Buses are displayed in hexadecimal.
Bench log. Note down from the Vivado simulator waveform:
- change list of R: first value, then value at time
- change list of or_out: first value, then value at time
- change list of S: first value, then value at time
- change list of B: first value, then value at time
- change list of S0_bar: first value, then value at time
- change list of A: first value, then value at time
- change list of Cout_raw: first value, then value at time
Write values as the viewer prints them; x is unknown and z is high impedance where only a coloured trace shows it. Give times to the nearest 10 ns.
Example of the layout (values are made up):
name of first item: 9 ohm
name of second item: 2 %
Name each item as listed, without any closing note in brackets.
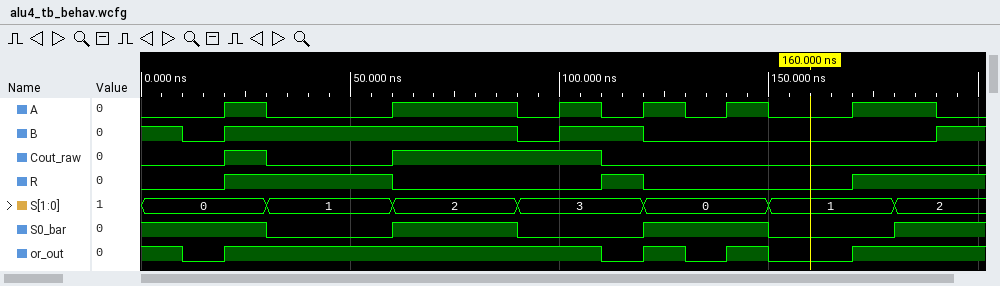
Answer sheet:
change list of R: first value, then value at time: 0, 1 at 20 ns, 0 at 60 ns, 1 at 110 ns, 0 at 120 ns, 1 at 170 ns
change list of or_out: first value, then value at time: 1, 0 at 10 ns, 1 at 20 ns, 0 at 110 ns, 1 at 120 ns, 0 at 130 ns, 1 at 140 ns, 0 at 150 ns, 1 at 170 ns
change list of S: first value, then value at time: 0, 1 at 30 ns, 2 at 60 ns, 3 at 90 ns, 0 at 120 ns, 1 at 150 ns, 2 at 180 ns
change list of B: first value, then value at time: 1, 0 at 10 ns, 1 at 20 ns, 0 at 90 ns, 1 at 100 ns, 0 at 120 ns, 1 at 190 ns
change list of S0_bar: first value, then value at time: 1, 0 at 30 ns, 1 at 60 ns, 0 at 90 ns, 1 at 120 ns, 0 at 150 ns, 1 at 180 ns
change list of A: first value, then value at time: 0, 1 at 20 ns, 0 at 30 ns, 1 at 60 ns, 0 at 90 ns, 1 at 100 ns, 0 at 110 ns, 1 at 120 ns, 0 at 130 ns, 1 at 140 ns, 0 at 150 ns, 1 at 170 ns, 0 at 190 ns
change list of Cout_raw: first value, then value at time: 0, 1 at 20 ns, 0 at 30 ns, 1 at 60 ns, 0 at 110 ns
